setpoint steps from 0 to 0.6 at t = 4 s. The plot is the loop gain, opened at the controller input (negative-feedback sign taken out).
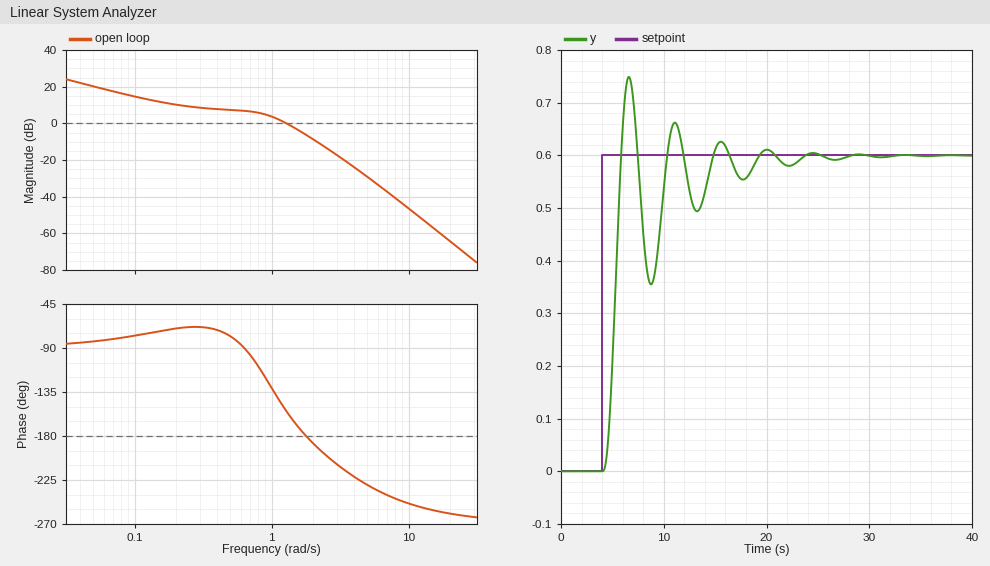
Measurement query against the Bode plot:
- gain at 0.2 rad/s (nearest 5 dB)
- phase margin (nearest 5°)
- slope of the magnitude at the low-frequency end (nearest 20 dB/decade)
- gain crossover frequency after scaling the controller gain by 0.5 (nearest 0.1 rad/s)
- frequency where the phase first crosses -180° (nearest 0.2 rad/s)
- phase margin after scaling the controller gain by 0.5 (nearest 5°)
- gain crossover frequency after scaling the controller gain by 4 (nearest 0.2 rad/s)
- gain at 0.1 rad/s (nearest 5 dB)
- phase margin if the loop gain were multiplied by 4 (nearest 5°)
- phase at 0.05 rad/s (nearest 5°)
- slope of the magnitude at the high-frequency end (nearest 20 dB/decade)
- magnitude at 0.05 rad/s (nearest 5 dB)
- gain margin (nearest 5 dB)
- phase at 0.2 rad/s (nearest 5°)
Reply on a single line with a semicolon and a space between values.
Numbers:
10 dB; 25°; -20 dB/decade; 0.8 rad/s; 1.8 rad/s; 75°; 2.4 rad/s; 15 dB; -15°; -85°; -60 dB/decade; 20 dB; 5 dB; -70°
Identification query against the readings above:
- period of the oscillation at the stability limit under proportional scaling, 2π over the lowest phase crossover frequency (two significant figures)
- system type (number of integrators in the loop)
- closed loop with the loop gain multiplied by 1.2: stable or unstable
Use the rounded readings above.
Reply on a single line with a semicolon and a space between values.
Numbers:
3.5 s; 1; stable
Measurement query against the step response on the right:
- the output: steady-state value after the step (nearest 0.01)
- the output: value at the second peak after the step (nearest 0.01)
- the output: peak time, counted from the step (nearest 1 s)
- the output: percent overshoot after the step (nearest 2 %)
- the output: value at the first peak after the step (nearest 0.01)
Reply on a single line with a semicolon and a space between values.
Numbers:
0.60; 0.66; 3 s; 24 %; 0.75
